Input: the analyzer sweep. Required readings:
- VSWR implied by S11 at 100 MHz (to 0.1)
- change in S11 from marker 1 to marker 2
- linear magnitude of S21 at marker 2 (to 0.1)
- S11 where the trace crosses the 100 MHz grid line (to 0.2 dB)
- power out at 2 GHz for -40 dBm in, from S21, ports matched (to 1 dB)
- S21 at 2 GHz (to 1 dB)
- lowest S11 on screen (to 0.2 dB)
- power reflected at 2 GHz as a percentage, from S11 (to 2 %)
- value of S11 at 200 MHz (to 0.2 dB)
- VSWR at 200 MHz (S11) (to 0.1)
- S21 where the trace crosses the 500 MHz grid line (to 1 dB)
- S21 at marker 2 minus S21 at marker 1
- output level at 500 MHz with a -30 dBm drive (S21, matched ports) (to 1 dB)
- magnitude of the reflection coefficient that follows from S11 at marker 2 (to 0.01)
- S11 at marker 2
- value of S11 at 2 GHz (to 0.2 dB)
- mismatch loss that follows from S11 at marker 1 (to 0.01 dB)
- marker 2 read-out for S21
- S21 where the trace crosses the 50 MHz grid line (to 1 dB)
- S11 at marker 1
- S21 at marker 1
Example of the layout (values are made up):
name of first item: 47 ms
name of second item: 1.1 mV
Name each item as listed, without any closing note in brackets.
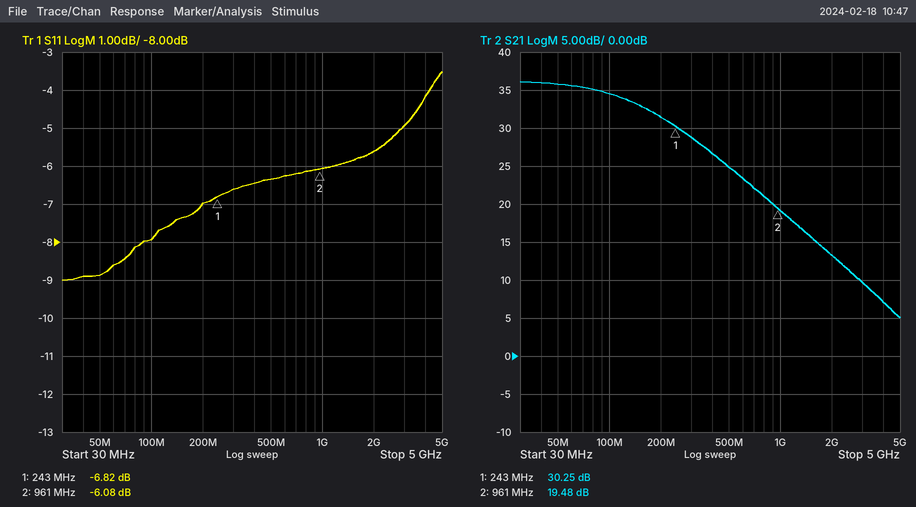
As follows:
VSWR implied by S11 at 100 MHz: 2.3
change in S11 from marker 1 to marker 2: 0.74 dB
linear magnitude of S21 at marker 2: 9.4
S11 where the trace crosses the 100 MHz grid line: -8.0 dB
power out at 2 GHz for -40 dBm in, from S21, ports matched: -27 dBm
S21 at 2 GHz: 13 dB
lowest S11 on screen: -9.0 dB
power reflected at 2 GHz as a percentage, from S11: 28 %
value of S11 at 200 MHz: -7.0 dB
VSWR at 200 MHz (S11): 2.6
S21 where the trace crosses the 500 MHz grid line: 25 dB
S21 at marker 2 minus S21 at marker 1: -10.77 dB
output level at 500 MHz with a -30 dBm drive (S21, matched ports): -5 dBm
magnitude of the reflection coefficient that follows from S11 at marker 2: 0.50
S11 at marker 2: -6.08 dB
value of S11 at 2 GHz: -5.6 dB
mismatch loss that follows from S11 at marker 1: 1.01 dB
marker 2 read-out for S21: 19.48 dB
S21 where the trace crosses the 50 MHz grid line: 36 dB
S11 at marker 1: -6.82 dB
S21 at marker 1: 30.25 dB
